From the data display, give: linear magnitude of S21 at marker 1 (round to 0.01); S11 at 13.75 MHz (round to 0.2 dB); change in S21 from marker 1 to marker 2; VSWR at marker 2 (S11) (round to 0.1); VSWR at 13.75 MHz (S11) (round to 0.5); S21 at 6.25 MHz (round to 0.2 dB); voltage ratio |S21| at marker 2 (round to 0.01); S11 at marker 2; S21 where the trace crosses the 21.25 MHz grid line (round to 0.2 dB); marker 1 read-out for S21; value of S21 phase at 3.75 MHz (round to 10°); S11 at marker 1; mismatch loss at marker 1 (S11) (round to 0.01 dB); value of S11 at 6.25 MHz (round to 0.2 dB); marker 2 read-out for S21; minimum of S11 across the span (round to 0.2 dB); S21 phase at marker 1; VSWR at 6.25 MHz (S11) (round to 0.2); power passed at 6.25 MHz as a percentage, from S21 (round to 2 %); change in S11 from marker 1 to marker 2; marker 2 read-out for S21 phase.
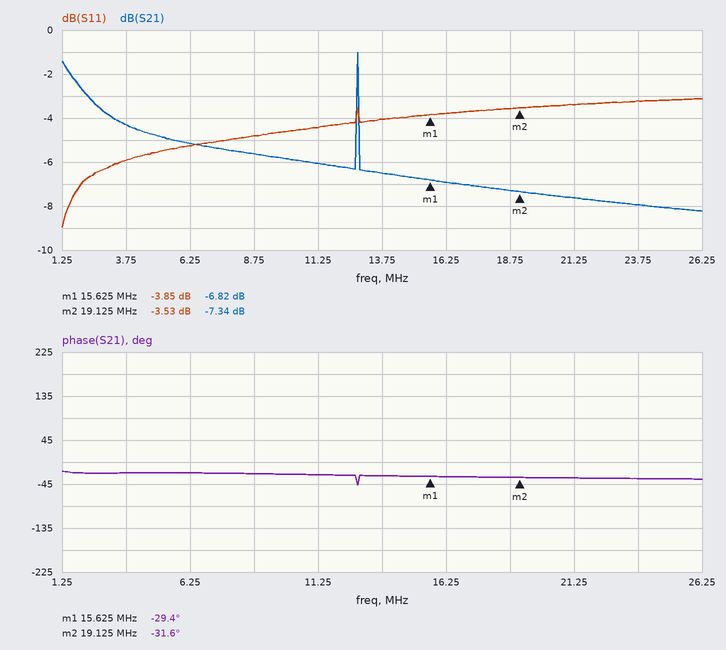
0.46
-4.0 dB
-0.52 dB
5.0
4.5
-5.2 dB
0.43
-3.53 dB
-7.6 dB
-6.82 dB
-20°
-3.85 dB
2.31 dB
-5.2 dB
-7.34 dB
-9.0 dB
-29.4°
3.4
30 %
0.32 dB
-31.6°
